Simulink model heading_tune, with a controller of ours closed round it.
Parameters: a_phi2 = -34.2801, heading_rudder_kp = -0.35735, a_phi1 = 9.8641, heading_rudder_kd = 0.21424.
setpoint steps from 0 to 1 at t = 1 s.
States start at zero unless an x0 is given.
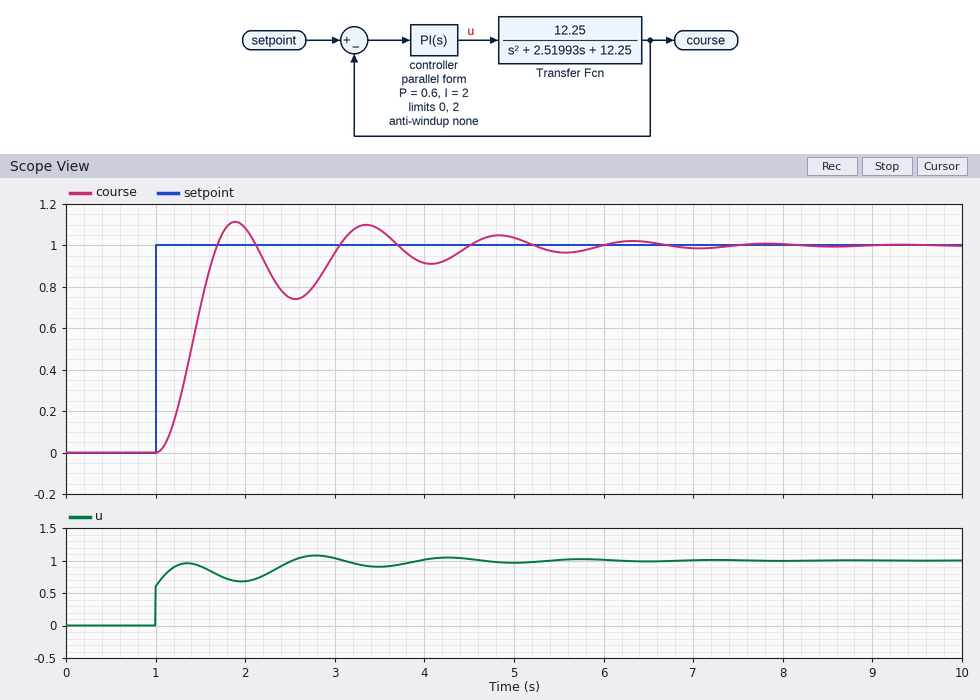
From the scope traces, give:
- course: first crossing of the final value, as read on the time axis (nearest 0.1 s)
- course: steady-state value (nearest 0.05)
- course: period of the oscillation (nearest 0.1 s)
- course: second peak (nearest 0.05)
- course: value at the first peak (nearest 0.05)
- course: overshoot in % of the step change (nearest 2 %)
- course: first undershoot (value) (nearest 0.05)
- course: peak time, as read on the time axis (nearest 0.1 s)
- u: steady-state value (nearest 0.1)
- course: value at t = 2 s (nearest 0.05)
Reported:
1.7 s
1.00
1.5 s
1.10
1.10
12 %
0.75
1.9 s
1.0
1.10
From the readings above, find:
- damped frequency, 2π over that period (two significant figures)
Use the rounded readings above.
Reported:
4.2 rad/s
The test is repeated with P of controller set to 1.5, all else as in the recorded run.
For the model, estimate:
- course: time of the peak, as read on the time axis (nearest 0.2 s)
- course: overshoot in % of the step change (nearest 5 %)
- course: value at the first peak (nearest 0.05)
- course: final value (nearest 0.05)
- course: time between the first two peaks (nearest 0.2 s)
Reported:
1.6 s
15 %
1.15
1.00
1.2 s
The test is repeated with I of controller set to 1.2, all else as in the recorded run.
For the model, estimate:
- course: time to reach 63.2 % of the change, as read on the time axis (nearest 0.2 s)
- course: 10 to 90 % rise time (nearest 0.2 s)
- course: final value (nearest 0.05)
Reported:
1.6 s
1.8 s
1.00
